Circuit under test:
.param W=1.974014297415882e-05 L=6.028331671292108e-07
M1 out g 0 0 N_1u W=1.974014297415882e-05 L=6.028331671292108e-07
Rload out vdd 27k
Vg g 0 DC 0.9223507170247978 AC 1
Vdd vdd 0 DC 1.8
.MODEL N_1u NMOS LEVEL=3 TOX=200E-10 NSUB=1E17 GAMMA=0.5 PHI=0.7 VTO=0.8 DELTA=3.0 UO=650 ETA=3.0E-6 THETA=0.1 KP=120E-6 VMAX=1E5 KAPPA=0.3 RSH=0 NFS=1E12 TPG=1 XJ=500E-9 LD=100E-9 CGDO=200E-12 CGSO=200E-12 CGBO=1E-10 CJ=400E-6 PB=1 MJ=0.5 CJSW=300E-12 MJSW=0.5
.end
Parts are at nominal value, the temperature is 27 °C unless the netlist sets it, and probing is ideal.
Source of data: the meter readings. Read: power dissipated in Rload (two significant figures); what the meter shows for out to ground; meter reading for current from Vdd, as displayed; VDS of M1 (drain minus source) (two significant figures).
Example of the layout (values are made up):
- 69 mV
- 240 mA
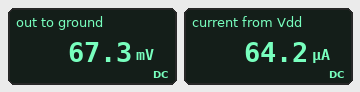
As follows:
- 110 µW
- 67.3 mV
- 64.2 µA
- 67 mV
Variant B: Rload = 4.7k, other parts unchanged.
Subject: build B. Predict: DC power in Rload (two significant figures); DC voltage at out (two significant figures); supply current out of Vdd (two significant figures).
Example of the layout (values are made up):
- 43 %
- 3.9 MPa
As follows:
- 58 µW
- 1.3 V
- 110 µA
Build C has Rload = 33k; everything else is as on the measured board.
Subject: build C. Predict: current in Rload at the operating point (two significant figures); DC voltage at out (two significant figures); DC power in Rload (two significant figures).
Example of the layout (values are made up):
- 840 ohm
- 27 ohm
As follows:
- 53 µA
- 52 mV
- 93 µW
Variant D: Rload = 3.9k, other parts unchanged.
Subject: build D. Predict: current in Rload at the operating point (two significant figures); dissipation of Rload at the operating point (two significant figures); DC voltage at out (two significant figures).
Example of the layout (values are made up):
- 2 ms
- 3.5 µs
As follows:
- 110 µA
- 49 µW
- 1.4 V
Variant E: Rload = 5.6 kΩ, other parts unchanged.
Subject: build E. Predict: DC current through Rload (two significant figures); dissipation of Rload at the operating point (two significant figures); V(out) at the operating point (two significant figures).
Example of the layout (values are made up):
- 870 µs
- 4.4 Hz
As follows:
- 110 µA
- 68 µW
- 1.2 V
